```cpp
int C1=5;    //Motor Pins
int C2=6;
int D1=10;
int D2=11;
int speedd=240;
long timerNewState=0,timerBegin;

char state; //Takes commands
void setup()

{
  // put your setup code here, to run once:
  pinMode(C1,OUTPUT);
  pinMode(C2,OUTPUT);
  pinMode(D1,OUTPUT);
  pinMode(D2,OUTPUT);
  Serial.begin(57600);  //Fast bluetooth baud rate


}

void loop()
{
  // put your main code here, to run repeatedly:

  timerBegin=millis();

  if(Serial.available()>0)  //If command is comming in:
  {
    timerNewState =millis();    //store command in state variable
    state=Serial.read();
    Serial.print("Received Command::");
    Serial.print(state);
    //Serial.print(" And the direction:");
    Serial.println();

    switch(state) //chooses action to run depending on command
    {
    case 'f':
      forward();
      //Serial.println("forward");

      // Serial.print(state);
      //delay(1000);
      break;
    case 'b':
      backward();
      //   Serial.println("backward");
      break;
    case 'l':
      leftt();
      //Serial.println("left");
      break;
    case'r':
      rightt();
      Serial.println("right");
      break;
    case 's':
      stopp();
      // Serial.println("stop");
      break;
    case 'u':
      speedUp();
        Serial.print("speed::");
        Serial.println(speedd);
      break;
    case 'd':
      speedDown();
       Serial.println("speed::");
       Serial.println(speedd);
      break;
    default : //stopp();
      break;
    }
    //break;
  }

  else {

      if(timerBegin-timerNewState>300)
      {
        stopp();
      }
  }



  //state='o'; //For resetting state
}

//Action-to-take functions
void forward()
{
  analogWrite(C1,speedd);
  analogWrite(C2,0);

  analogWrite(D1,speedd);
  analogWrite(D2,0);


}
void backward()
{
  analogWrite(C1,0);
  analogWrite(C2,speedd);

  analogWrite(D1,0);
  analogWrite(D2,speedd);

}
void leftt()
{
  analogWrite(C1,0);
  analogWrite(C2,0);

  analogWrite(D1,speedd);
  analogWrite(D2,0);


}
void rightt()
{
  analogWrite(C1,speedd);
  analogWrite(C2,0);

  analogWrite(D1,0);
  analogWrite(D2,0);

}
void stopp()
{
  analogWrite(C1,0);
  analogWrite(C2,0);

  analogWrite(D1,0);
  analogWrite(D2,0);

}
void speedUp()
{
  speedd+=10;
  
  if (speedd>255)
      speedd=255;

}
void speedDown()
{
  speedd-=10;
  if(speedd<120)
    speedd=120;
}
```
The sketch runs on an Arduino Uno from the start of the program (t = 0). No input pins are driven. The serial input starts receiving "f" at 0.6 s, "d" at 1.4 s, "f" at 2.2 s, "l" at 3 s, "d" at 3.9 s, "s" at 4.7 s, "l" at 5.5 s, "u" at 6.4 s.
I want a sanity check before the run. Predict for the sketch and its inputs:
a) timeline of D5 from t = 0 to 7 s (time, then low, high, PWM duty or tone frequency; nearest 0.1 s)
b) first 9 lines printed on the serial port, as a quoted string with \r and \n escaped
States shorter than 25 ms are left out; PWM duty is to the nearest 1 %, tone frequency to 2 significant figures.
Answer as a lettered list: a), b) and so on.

a) 0 s low; 0.6 s PWM 94 %; 0.9 s low; 2.2 s PWM 90 %; 2.5 s low
b) "Received Command::f\r\nReceived Command::d\r\nspeed::\r\n230\r\nReceived Command::f\r\nReceived Command::l\r\nReceived Command::d\r\nspeed::\r\n220\r\n"
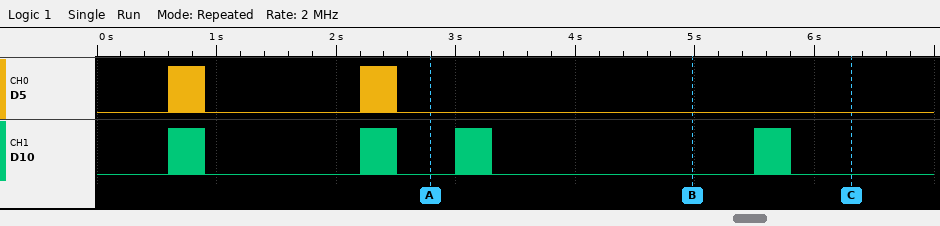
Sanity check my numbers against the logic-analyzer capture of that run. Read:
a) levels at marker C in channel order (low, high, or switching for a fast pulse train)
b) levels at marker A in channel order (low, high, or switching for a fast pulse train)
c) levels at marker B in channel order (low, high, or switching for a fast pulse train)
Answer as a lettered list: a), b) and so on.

a) D5 low, D10 low
b) D5 low, D10 low
c) D5 low, D10 low
